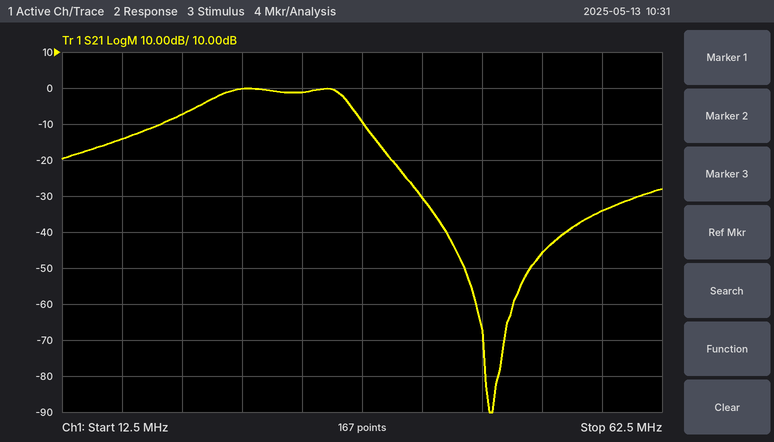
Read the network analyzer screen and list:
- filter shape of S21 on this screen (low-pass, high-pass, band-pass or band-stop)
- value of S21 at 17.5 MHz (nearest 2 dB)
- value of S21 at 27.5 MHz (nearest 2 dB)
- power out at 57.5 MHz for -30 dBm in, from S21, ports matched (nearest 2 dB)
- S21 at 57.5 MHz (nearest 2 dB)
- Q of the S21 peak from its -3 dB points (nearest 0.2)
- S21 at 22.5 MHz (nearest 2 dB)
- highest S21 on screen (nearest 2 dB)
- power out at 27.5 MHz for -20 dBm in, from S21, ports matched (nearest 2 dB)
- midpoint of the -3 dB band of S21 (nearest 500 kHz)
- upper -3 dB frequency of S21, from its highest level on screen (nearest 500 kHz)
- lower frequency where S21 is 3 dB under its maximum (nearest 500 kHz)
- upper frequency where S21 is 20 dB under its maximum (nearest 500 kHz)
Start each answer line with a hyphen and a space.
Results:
- band-pass
- -14 dB
- 0 dB
- -64 dBm
- -34 dB
- 2.8
- -8 dB
- 0 dB
- -20 dBm
- 30.5 MHz
- 36.0 MHz
- 25.0 MHz
- 40.0 MHz
